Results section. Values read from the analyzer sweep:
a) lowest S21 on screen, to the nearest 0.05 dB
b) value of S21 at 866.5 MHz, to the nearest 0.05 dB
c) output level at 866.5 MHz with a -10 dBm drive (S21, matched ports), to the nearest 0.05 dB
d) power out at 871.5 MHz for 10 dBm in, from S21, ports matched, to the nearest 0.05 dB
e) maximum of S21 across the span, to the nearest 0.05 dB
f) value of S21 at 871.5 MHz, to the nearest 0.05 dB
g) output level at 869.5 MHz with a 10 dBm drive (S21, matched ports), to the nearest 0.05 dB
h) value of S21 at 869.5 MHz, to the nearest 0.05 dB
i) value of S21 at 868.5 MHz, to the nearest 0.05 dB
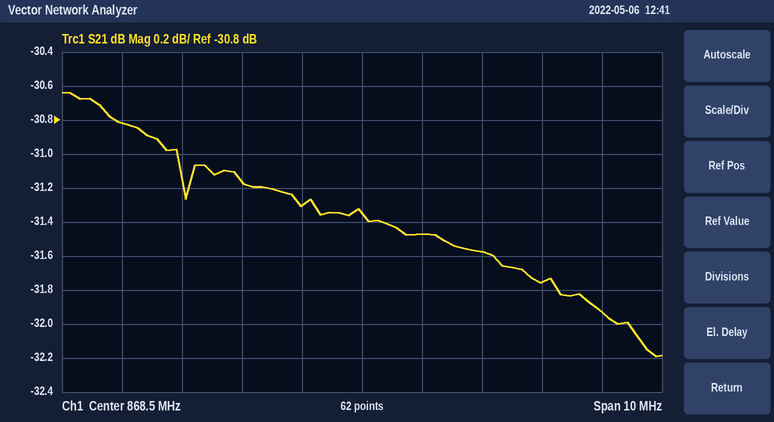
-32.20 dB
-31.15 dB
-41.15 dBm
-21.75 dBm
-30.65 dB
-31.75 dB
-21.45 dBm
-31.45 dB
-31.35 dB
